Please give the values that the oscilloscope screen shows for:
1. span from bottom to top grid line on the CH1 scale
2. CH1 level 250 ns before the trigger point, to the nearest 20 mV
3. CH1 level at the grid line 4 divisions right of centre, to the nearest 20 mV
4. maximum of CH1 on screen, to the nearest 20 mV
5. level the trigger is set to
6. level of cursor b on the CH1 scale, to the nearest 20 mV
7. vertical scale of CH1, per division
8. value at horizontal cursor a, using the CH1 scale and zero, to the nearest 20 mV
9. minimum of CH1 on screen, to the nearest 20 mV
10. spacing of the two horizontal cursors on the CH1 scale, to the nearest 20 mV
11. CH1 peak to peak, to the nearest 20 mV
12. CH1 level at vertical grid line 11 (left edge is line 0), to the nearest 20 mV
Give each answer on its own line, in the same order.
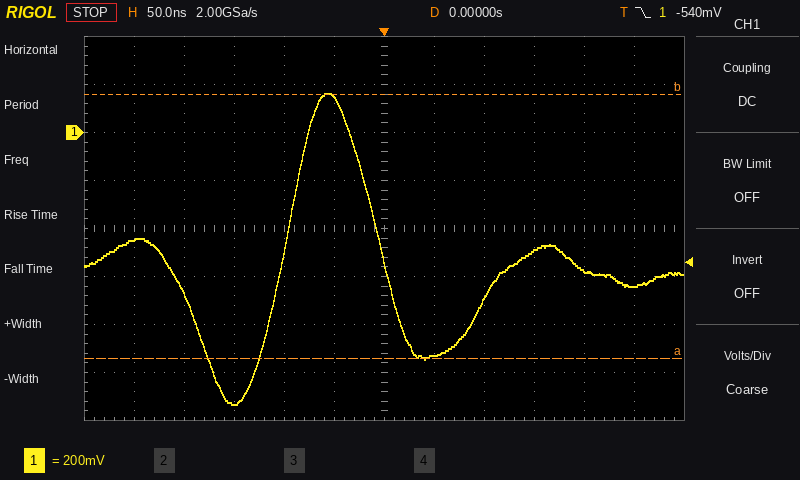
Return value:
1.6 V
-440 mV
-580 mV
160 mV
-540 mV
160 mV
200 mV
-940 mV
-1.14 V
1.10 V
1.30 V
-640 mV
